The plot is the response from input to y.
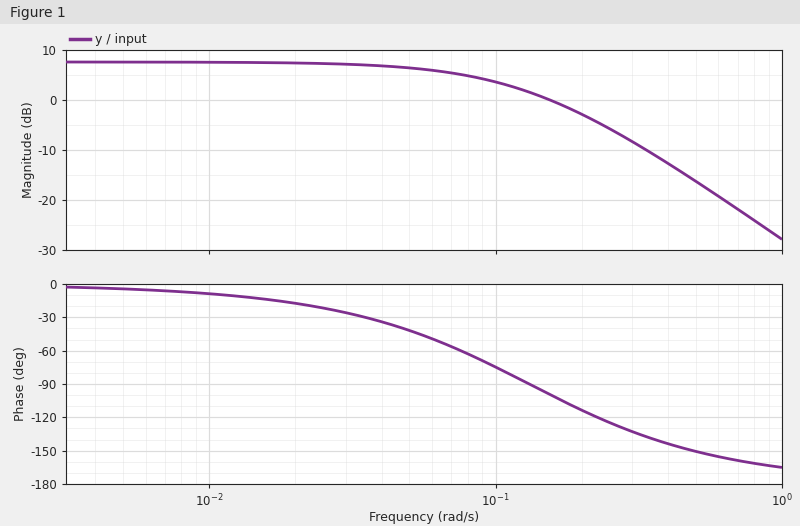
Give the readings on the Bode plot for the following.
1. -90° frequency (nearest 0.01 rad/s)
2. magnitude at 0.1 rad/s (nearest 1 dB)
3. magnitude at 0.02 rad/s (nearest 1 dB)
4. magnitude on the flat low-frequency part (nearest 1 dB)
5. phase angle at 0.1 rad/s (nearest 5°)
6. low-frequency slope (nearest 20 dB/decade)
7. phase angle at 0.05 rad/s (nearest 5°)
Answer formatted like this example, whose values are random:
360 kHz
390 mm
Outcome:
0.13 rad/s
4 dB
7 dB
8 dB
-75°
0 dB/decade
-40°
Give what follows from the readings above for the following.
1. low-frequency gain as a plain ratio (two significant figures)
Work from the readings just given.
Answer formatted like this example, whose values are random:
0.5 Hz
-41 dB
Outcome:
2.5
